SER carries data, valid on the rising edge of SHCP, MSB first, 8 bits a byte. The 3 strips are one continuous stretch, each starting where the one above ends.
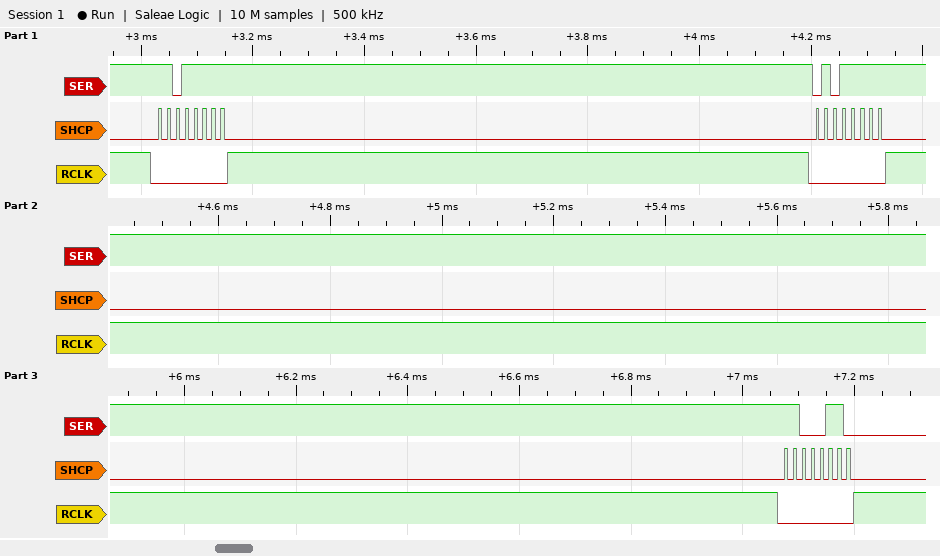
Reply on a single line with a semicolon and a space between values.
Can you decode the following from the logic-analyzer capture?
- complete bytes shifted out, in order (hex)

0xDF 0x5F 0xC6
